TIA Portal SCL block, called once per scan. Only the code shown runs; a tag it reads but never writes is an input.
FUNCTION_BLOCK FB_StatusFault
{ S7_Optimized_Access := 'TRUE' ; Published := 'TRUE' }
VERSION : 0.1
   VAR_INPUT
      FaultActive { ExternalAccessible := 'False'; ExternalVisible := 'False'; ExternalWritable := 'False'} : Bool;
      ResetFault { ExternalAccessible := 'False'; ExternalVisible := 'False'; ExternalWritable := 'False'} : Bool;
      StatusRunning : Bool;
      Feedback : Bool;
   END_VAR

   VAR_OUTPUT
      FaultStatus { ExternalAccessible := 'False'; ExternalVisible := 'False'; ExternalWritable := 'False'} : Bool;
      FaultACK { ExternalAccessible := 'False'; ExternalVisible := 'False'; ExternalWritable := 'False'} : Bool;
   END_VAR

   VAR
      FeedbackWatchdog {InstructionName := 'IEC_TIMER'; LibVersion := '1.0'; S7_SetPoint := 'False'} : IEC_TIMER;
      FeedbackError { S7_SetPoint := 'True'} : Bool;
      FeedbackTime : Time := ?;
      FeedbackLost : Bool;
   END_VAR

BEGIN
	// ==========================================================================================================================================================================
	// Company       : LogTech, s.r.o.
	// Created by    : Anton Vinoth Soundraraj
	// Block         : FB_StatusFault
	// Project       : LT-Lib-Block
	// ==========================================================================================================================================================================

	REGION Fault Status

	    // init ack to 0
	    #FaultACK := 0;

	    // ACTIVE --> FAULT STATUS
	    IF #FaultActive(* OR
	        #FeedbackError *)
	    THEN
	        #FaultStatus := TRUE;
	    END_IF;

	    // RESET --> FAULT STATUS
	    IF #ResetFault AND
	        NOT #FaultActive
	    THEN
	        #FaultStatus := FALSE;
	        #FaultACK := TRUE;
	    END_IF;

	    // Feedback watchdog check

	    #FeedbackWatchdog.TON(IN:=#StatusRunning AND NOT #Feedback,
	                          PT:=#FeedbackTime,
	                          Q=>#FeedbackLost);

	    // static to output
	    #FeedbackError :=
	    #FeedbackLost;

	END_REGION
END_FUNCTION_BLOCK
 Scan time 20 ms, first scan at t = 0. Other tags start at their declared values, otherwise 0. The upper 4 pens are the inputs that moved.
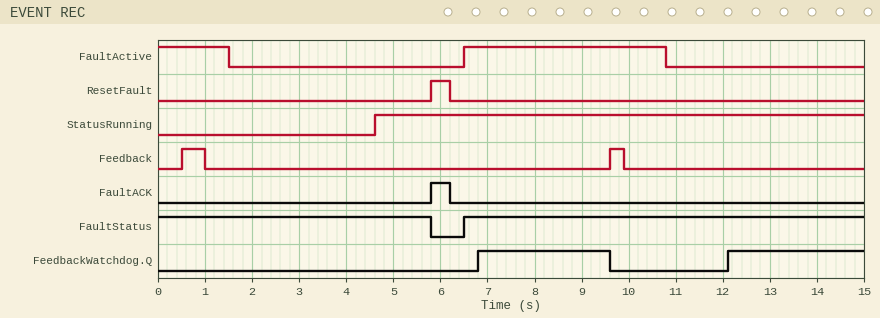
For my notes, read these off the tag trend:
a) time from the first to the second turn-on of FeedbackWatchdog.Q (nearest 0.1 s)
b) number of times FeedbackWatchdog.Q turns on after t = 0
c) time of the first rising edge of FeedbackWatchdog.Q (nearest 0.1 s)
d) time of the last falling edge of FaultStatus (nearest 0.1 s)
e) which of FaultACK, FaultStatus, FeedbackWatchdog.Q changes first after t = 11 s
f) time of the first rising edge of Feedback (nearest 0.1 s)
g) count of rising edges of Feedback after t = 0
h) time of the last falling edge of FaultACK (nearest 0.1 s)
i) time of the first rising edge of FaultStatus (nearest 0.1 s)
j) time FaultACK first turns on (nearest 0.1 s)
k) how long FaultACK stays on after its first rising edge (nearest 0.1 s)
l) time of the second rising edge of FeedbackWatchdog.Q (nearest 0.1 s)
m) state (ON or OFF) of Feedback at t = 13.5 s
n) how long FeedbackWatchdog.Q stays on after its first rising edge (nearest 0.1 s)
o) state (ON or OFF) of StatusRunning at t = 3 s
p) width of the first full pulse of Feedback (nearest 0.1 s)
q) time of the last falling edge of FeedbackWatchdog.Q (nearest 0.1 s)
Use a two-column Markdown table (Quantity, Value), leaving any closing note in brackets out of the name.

| Quantity | Value |
|---|---|
| time from the first to the second turn-on of FeedbackWatchdog.Q | 5.3 s |
| number of times FeedbackWatchdog.Q turns on after t = 0 | 2 |
| time of the first rising edge of FeedbackWatchdog.Q | 6.8 s |
| time of the last falling edge of FaultStatus | 5.8 s |
| which of FaultACK, FaultStatus, FeedbackWatchdog.Q changes first after t = 11 s | FeedbackWatchdog.Q |
| time of the first rising edge of Feedback | 0.5 s |
| count of rising edges of Feedback after t = 0 | 2 |
| time of the last falling edge of FaultACK | 6.2 s |
| time of the first rising edge of FaultStatus | 6.5 s |
| time FaultACK first turns on | 5.8 s |
| how long FaultACK stays on after its first rising edge | 0.4 s |
| time of the second rising edge of FeedbackWatchdog.Q | 12.1 s |
| state (ON or OFF) of Feedback at t = 13.5 s | OFF |
| how long FeedbackWatchdog.Q stays on after its first rising edge | 2.8 s |
| state (ON or OFF) of StatusRunning at t = 3 s | OFF |
| width of the first full pulse of Feedback | 0.5 s |
| time of the last falling edge of FeedbackWatchdog.Q | 9.6 s |
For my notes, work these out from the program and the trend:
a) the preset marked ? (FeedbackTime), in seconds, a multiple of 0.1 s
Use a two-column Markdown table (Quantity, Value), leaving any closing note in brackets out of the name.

| Quantity | Value |
|---|---|
| the preset marked ? (FeedbackTime), in seconds, a multiple of 0.1 s | 2.2 s |
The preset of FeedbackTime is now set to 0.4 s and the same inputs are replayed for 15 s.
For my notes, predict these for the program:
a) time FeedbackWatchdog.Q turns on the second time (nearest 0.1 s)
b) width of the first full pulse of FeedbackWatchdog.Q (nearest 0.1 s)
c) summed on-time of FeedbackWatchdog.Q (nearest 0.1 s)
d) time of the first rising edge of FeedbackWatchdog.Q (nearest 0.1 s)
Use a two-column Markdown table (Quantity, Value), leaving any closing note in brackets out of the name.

| Quantity | Value |
|---|---|
| time FeedbackWatchdog.Q turns on the second time | 10.3 s |
| width of the first full pulse of FeedbackWatchdog.Q | 4.6 s |
| summed on-time of FeedbackWatchdog.Q | 9.3 s |
| time of the first rising edge of FeedbackWatchdog.Q | 5.0 s |
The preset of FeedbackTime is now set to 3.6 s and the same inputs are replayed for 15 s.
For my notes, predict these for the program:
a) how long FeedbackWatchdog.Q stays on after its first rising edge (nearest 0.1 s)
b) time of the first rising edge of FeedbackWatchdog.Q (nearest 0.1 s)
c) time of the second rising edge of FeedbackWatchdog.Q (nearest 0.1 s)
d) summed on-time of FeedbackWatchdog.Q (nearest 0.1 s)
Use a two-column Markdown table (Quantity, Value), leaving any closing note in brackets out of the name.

| Quantity | Value |
|---|---|
| how long FeedbackWatchdog.Q stays on after its first rising edge | 1.4 s |
| time of the first rising edge of FeedbackWatchdog.Q | 8.2 s |
| time of the second rising edge of FeedbackWatchdog.Q | 13.5 s |
| summed on-time of FeedbackWatchdog.Q | 2.9 s |
